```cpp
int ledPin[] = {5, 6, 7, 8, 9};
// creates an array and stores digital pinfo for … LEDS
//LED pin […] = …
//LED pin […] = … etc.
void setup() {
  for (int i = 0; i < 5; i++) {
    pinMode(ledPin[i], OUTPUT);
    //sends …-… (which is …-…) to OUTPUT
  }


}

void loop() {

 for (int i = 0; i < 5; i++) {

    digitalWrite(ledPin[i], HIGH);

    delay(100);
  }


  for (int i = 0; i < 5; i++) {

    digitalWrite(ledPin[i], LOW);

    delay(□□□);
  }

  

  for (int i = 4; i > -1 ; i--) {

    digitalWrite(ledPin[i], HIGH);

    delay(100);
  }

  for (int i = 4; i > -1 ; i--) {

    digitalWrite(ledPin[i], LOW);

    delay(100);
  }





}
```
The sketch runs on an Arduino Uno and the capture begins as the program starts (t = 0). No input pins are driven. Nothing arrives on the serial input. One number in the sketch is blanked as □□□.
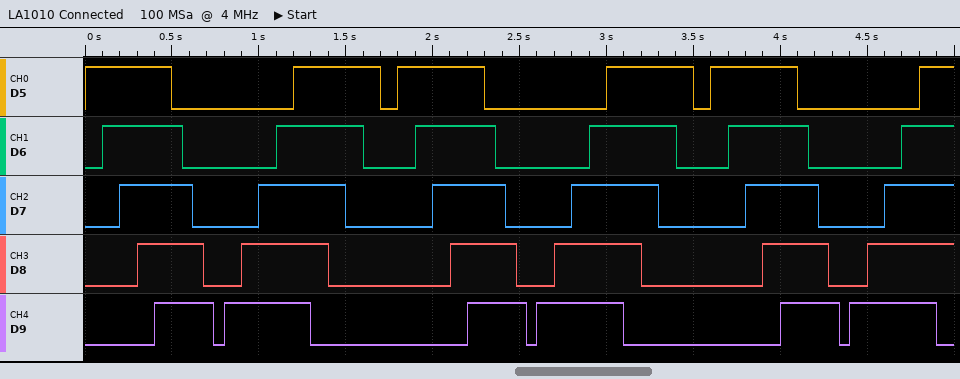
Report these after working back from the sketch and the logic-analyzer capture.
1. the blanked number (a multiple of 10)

60
